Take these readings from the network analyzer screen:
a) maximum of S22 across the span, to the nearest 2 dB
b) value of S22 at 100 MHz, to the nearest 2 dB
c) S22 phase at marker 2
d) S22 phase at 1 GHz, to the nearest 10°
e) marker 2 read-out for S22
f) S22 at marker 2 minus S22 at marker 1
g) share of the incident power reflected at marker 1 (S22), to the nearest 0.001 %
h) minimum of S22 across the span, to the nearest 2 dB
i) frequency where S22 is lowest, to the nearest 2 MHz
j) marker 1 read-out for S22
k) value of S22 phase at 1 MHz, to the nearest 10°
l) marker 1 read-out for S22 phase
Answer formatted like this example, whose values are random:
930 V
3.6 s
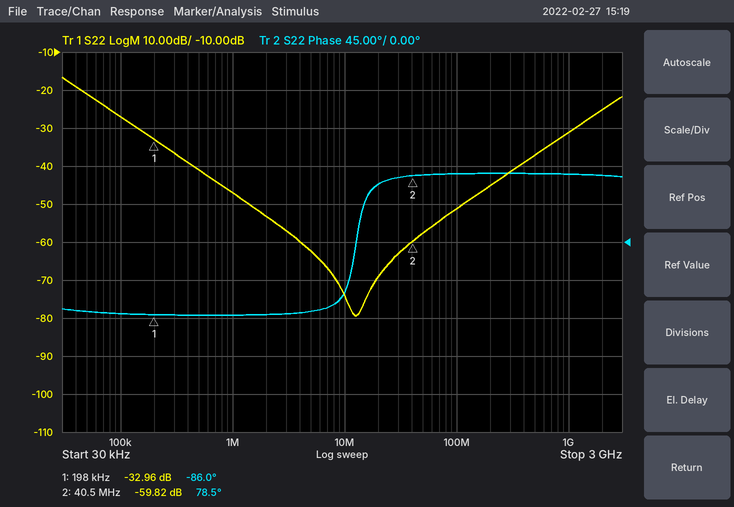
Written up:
-16 dB
-52 dB
78.5°
80°
-59.82 dB
-26.86 dB
0.051 %
-80 dB
12 MHz
-32.96 dB
-90°
-86.0°
